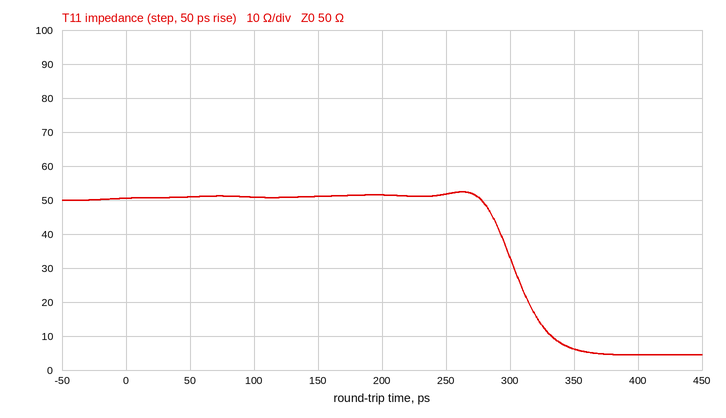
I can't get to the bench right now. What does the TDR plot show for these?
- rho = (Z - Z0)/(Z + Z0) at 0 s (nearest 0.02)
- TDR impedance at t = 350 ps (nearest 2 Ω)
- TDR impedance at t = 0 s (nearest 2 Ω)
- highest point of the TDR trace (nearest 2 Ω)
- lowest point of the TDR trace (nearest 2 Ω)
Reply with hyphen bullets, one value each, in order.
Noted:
- 0.00
- 6 Ω
- 50 Ω
- 52 Ω
- 4 Ω
